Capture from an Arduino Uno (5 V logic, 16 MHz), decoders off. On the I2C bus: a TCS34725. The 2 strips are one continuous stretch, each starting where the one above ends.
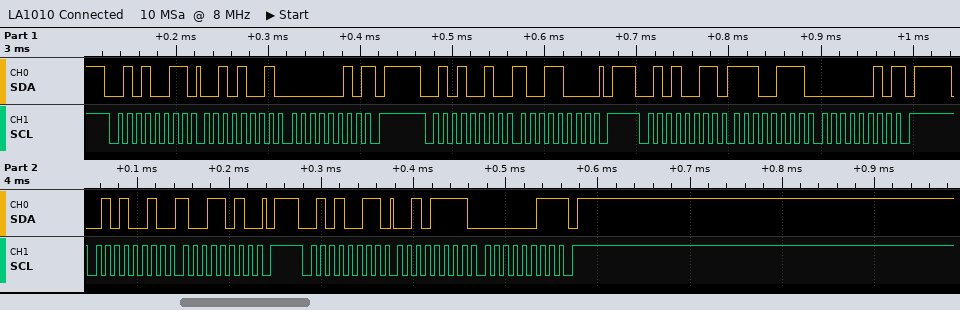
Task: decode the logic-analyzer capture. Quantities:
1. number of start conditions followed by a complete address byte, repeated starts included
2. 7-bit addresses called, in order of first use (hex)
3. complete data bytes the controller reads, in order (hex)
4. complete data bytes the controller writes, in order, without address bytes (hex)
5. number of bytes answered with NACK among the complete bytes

5
0x29
29 02 E7 02 2F 03
98 9A
3
